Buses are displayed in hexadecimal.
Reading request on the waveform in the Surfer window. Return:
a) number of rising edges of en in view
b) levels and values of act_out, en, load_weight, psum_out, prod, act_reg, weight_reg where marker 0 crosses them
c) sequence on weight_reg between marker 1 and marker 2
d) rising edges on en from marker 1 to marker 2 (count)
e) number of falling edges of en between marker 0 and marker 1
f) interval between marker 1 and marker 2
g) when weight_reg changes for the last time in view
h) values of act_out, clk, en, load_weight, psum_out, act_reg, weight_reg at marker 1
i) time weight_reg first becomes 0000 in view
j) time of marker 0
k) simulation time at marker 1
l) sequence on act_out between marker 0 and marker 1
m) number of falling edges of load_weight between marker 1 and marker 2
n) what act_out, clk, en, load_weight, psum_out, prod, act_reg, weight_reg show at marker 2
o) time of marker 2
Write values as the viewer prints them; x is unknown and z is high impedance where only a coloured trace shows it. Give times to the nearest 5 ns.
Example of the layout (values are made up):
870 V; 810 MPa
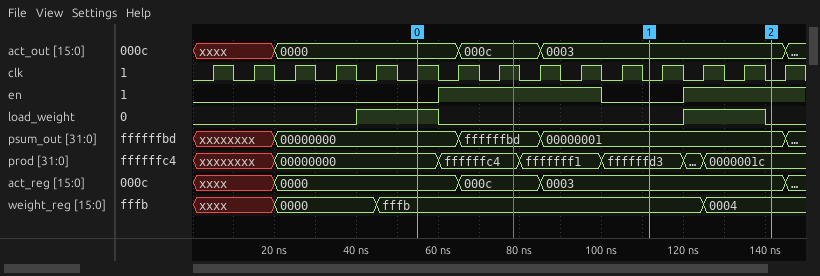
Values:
2; act_out=0000, en=0, load_weight=1, psum_out=00000000, prod=00000000, act_reg=0000, weight_reg=fffb; fffb, 0004; 1; 1; 30 ns; 125 ns; act_out=0003, clk=0, en=0, load_weight=0, psum_out=00000001, act_reg=0003, weight_reg=fffb; 20 ns; 55 ns; 110 ns; 0000, 000c, 0003; 1; act_out=0003, clk=0, en=1, load_weight=0, psum_out=00000001, prod=0000001c, act_reg=0003, weight_reg=0004; 140 ns
